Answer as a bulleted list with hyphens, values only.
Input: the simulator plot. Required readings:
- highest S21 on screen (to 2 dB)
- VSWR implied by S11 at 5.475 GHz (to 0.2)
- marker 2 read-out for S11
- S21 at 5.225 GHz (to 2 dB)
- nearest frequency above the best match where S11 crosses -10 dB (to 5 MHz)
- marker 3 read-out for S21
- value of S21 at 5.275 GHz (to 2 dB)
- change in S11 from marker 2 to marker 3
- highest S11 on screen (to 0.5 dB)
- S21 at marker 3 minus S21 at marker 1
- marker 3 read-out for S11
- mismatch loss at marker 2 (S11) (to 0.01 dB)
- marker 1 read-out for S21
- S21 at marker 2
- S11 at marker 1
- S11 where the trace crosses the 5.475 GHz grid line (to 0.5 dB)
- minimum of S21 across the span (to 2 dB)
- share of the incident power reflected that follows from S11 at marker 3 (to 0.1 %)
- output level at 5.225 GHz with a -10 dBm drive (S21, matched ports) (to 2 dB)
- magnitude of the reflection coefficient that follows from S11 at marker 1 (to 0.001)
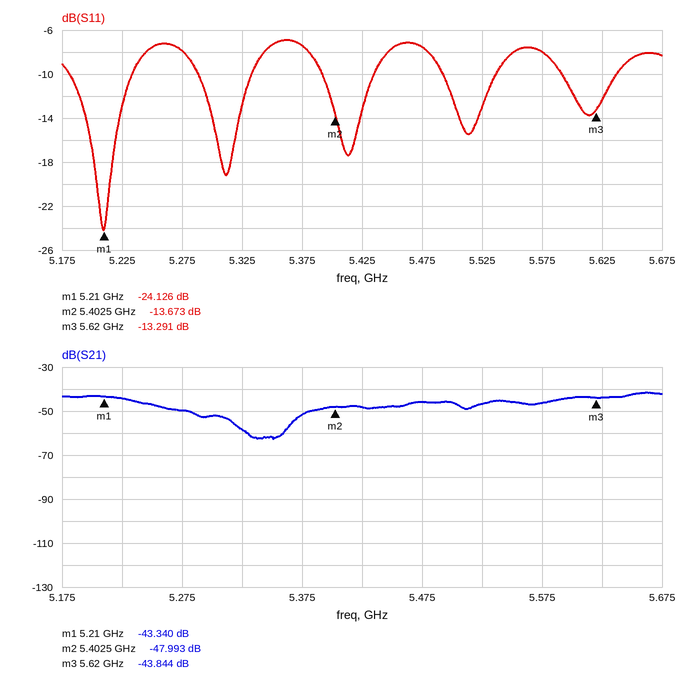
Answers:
- -42 dB
- 2.4
- -13.673 dB
- -44 dB
- 5.235 GHz
- -43.844 dB
- -50 dB
- 0.382 dB
- -7.0 dB
- -0.504 dB
- -13.291 dB
- 0.19 dB
- -43.340 dB
- -47.993 dB
- -24.126 dB
- -7.5 dB
- -62 dB
- 4.7 %
- -54 dBm
- 0.062
